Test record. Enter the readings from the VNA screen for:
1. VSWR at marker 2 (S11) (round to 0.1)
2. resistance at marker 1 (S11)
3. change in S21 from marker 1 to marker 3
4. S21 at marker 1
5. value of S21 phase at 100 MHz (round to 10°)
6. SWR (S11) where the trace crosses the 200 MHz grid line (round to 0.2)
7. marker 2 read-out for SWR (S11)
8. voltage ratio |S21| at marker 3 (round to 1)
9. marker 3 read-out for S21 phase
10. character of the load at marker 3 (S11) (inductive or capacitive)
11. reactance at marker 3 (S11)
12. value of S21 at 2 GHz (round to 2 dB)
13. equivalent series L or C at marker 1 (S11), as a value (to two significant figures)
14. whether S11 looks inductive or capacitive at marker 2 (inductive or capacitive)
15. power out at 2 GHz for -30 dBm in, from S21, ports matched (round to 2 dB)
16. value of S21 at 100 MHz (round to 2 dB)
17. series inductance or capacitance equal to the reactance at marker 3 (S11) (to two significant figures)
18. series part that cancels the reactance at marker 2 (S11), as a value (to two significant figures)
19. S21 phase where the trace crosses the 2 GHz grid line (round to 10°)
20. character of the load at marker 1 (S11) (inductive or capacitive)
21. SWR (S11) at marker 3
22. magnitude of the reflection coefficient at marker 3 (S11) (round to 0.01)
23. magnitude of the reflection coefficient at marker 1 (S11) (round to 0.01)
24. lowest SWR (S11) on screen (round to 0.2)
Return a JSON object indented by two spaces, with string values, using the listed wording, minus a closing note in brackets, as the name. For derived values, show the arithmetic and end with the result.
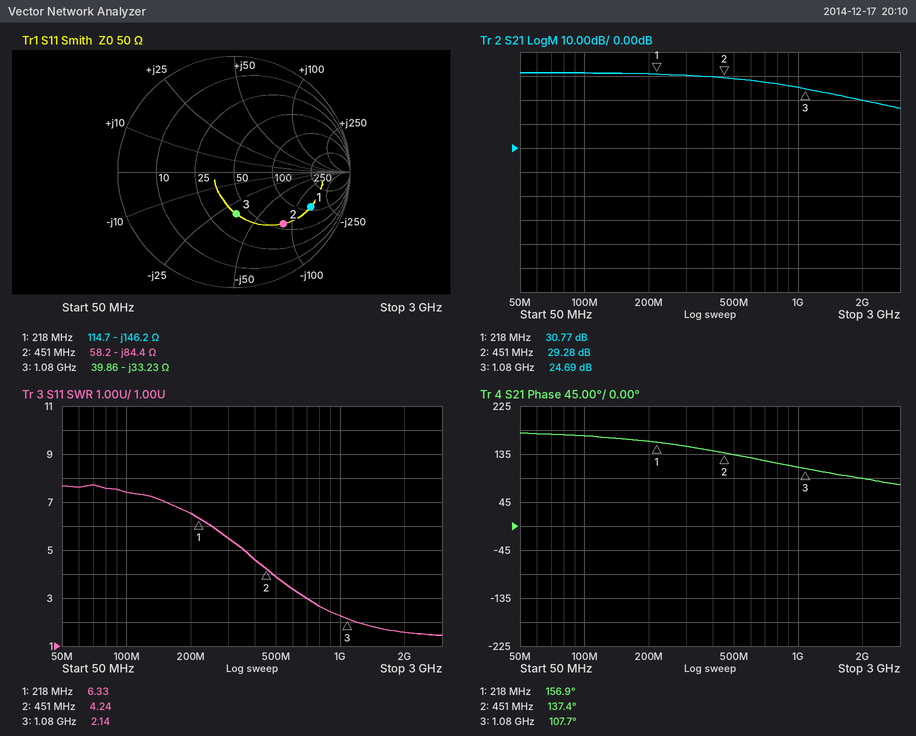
{
  "VSWR at marker 2 (S11)": "4.2",
  "resistance at marker 1": "114.7 Ω",
  "change in S21 from marker 1 to marker 3": "24.69 − (30.77) = -6.08 dB",
  "S21 at marker 1": "30.77 dB",
  "value of S21 phase at 100 MHz": "170°",
  "SWR (S11) where the trace crosses the 200 MHz grid line": "6.6",
  "marker 2 read-out for SWR": "4.24",
  "voltage ratio |S21| at marker 3": "10^(24.69/20) ≈ 17",
  "marker 3 read-out for S21 phase": "107.7°",
  "character of the load at marker 3 (S11)": "capacitive",
  "reactance at marker 3": "-33.23 Ω",
  "value of S21 at 2 GHz": "20 dB",
  "equivalent series L or C at marker 1 (S11), as a value": "C = 1/(2π × 218 MHz × 146.2 Ω) ≈ 5.0 pF",
  "whether S11 looks inductive or capacitive at marker 2": "capacitive",
  "power out at 2 GHz for -30 dBm in, from S21, ports matched": "-30 dBm + (20 dB) = -10 dBm",
  "value of S21 at 100 MHz": "32 dB",
  "series inductance or capacitance equal to the reactance at marker 3 (S11)": "C = 1/(2π × 1.08 GHz × 33.23 Ω) ≈ 4.4 pF",
  "series part that cancels the reactance at marker 2 (S11), as a value": "L = 84.4 Ω/(2π × 451 MHz) ≈ 30 nH",
  "S21 phase where the trace crosses the 2 GHz grid line": "90°",
  "character of the load at marker 1 (S11)": "capacitive",
  "SWR (S11) at marker 3": "2.14",
  "magnitude of the reflection coefficient at marker 3 (S11)": "0.36",
  "magnitude of the reflection coefficient at marker 1 (S11)": "0.73",
  "lowest SWR (S11) on screen": "1.4"
}
